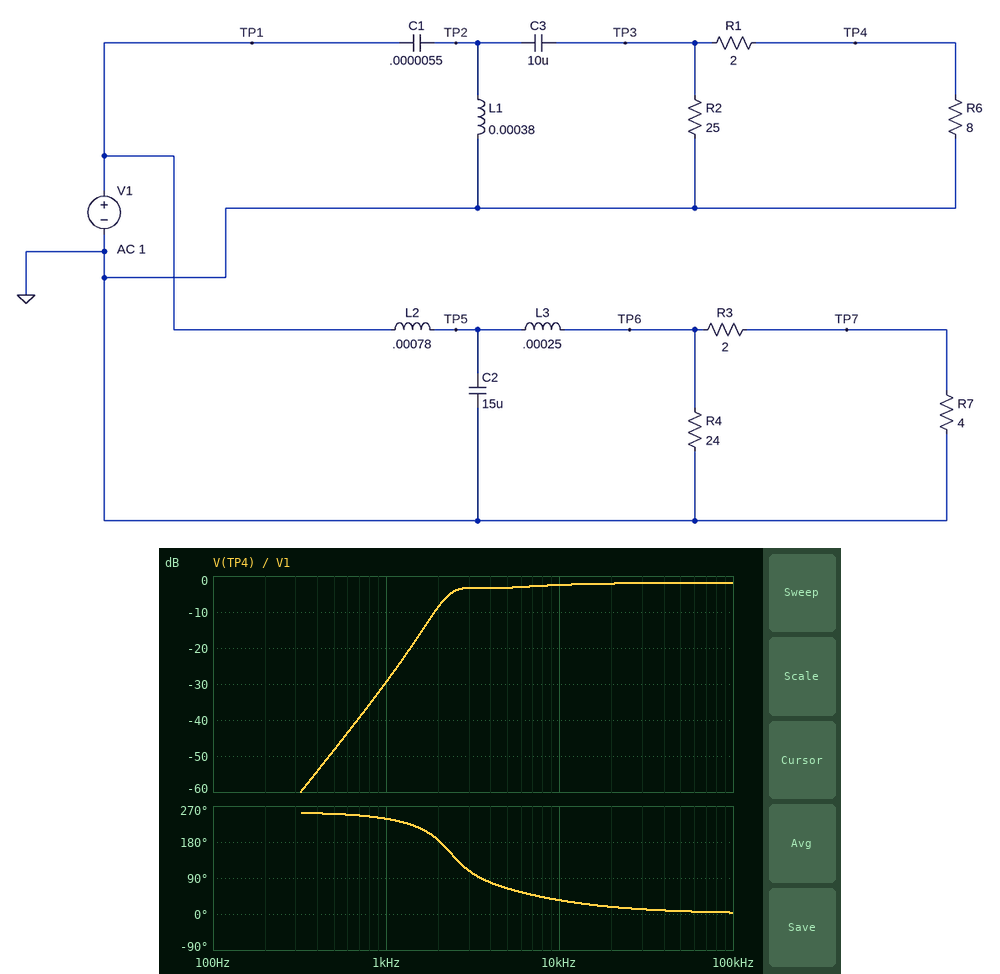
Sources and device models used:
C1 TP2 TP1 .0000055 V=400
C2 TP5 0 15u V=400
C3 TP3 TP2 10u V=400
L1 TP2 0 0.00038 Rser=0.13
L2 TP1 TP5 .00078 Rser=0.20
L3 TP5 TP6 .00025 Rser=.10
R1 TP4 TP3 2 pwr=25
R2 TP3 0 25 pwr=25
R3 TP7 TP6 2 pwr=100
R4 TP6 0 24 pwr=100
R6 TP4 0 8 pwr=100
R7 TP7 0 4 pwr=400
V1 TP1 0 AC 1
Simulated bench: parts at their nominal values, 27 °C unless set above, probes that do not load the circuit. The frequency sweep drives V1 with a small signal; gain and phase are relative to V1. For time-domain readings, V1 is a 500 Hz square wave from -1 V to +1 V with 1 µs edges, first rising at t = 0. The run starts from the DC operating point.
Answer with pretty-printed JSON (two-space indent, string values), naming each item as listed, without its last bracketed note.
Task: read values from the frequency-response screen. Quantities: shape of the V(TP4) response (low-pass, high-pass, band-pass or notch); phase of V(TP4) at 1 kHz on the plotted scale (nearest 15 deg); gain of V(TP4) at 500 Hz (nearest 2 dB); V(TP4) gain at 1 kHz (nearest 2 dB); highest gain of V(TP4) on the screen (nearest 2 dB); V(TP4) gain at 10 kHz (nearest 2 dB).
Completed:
{
  "shape of the V(TP4) response": "high-pass",
  "phase of V(TP4) at 1 kHz on the plotted scale": "240 deg",
  "gain of V(TP4) at 500 Hz": "-48 dB",
  "V(TP4) gain at 1 kHz": "-30 dB",
  "highest gain of V(TP4) on the screen": "-2 dB",
  "V(TP4) gain at 10 kHz": "-2 dB"
}
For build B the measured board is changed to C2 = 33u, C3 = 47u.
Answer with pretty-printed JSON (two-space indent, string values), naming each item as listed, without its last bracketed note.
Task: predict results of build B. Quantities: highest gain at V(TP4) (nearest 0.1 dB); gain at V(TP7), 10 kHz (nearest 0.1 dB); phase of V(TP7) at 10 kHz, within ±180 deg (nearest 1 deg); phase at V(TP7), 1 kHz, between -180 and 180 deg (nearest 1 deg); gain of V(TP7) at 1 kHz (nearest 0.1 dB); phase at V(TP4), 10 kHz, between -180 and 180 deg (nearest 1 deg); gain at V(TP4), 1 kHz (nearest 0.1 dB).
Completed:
{
  "highest gain at V(TP4)": "-1.8 dB",
  "gain at V(TP7), 10 kHz": "-54.0 dB",
  "phase of V(TP7) at 10 kHz, within ±180 deg": "108 deg",
  "phase at V(TP7), 1 kHz, between -180 and 180 deg": "-89 deg",
  "gain of V(TP7) at 1 kHz": "-4.0 dB",
  "phase at V(TP4), 10 kHz, between -180 and 180 deg": "27 deg",
  "gain at V(TP4), 1 kHz": "-23.1 dB"
}
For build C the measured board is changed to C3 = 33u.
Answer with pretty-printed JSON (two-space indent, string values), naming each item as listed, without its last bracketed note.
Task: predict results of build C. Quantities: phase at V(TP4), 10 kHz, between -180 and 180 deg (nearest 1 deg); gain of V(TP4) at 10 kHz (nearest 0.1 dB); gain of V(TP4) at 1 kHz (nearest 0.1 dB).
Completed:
{
  "phase at V(TP4), 10 kHz, between -180 and 180 deg": "28 deg",
  "gain of V(TP4) at 10 kHz": "-1.9 dB",
  "gain of V(TP4) at 1 kHz": "-23.4 dB"
}
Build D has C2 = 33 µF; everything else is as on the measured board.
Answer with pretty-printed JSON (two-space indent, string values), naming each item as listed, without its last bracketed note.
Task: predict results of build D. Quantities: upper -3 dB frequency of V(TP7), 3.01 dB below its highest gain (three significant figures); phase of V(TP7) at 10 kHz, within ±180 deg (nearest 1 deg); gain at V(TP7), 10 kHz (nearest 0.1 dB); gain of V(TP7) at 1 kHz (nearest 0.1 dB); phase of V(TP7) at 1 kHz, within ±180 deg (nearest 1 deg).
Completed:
{
  "upper -3 dB frequency of V(TP7), 3.01 dB below its highest gain": "1.40 kHz",
  "phase of V(TP7) at 10 kHz, within ±180 deg": "108 deg",
  "gain at V(TP7), 10 kHz": "-54.0 dB",
  "gain of V(TP7) at 1 kHz": "-4.0 dB",
  "phase of V(TP7) at 1 kHz, within ±180 deg": "-89 deg"
}
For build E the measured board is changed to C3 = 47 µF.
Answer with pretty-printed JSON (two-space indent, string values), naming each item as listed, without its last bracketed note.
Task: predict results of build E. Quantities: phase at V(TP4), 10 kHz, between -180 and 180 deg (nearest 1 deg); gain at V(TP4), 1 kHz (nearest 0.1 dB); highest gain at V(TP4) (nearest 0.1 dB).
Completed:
{
  "phase at V(TP4), 10 kHz, between -180 and 180 deg": "27 deg",
  "gain at V(TP4), 1 kHz": "-23.1 dB",
  "highest gain at V(TP4)": "-1.8 dB"
}
